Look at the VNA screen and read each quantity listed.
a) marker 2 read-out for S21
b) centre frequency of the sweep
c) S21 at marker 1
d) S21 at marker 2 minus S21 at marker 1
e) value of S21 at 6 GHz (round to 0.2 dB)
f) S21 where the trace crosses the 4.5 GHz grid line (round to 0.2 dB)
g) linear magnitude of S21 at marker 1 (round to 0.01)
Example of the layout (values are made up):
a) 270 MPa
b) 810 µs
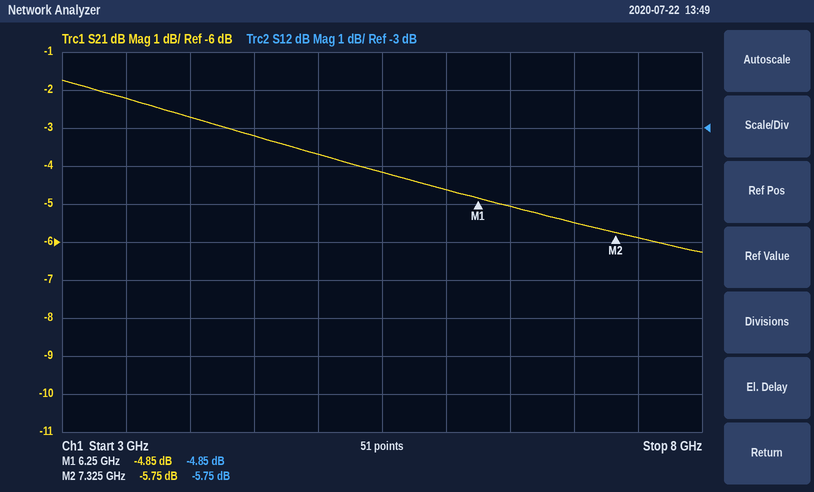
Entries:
a) -5.75 dB
b) 5.5 GHz
c) -4.85 dB
d) -0.90 dB
e) -4.6 dB
f) -3.2 dB
g) 0.57
